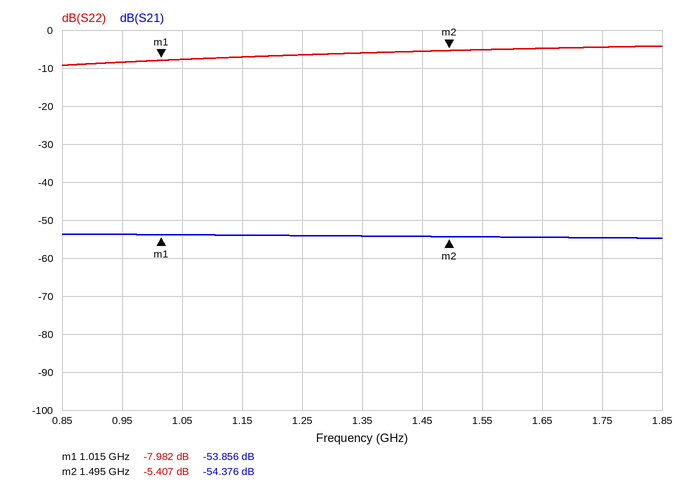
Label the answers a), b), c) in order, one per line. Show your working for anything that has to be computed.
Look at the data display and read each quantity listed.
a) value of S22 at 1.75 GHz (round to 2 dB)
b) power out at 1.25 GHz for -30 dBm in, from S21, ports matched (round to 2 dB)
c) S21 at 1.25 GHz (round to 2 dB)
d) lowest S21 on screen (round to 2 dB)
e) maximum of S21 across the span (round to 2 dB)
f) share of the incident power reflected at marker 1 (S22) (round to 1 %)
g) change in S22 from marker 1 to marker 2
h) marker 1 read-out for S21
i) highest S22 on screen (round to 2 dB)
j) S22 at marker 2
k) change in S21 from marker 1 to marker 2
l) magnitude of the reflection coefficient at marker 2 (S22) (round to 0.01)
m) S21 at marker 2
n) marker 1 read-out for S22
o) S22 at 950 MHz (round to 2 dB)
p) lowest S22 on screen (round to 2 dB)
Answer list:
a) -4 dB
b) -30 dBm + (-54 dB) = -84 dBm
c) -54 dB
d) -54 dB
e) -54 dB
f) 10^(-7.982/10) ≈ 16 %
g) -5.407 − (-7.982) = 2.575 dB
h) -53.856 dB
i) -4 dB
j) -5.407 dB
k) -54.376 − (-53.856) = -0.520 dB
l) 10^(-5.407/20) ≈ 0.54
m) -54.376 dB
n) -7.982 dB
o) -8 dB
p) -10 dB
